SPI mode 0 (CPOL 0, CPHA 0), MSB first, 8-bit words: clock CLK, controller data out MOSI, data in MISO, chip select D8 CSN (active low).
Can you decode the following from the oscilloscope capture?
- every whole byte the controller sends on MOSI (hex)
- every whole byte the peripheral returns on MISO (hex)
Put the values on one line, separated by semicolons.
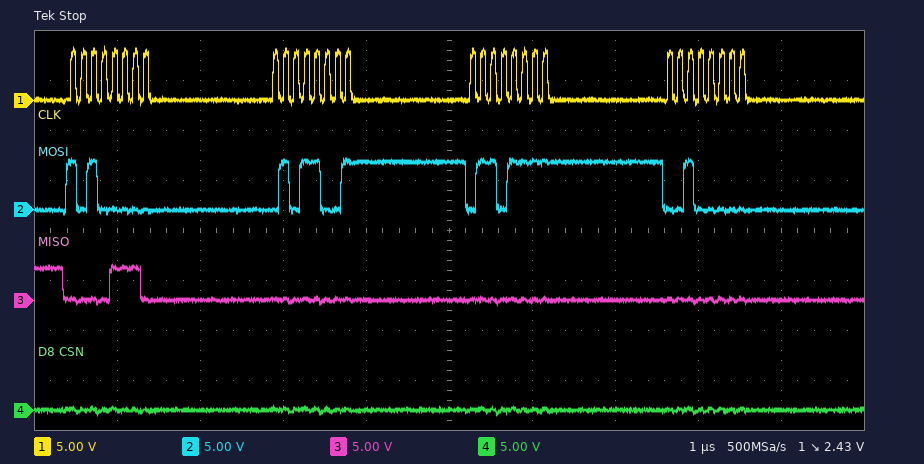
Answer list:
A0 59 6F 20; 0E 00 00 00
